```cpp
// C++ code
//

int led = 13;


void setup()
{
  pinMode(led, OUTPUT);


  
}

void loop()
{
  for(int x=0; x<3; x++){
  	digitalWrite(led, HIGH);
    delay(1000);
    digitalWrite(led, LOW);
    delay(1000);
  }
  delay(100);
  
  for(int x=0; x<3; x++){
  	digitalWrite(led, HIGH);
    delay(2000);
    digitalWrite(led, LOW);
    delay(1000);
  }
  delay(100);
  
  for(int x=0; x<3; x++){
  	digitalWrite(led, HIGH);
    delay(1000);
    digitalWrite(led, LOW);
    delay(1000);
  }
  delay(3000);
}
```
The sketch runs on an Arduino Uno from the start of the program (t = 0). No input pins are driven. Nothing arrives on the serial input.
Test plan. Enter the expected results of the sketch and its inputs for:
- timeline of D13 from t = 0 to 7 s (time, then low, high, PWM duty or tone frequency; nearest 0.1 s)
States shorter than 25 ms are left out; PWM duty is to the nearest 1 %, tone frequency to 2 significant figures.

0 s high; 1 s low; 2 s high; 3 s low; 4 s high; 5 s low; 6.1 s high
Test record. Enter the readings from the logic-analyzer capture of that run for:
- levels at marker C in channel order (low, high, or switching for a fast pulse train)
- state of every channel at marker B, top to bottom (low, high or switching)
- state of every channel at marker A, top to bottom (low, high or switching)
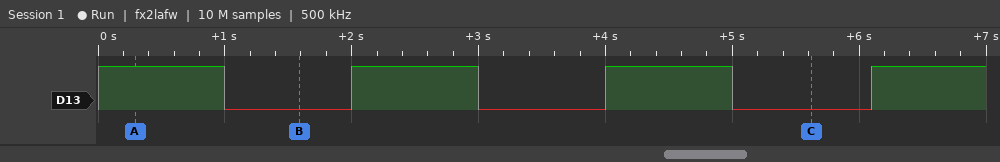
D13 low
D13 low
D13 high
